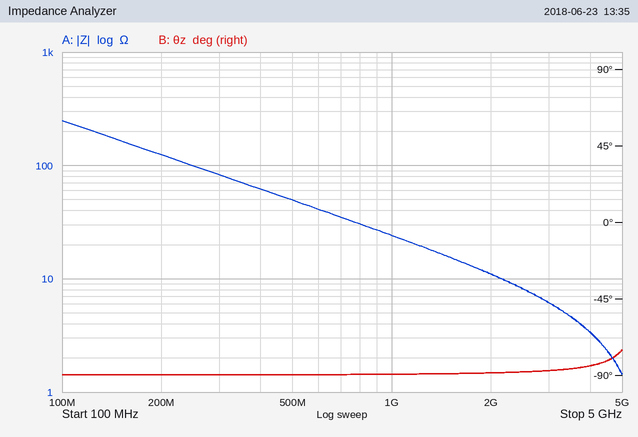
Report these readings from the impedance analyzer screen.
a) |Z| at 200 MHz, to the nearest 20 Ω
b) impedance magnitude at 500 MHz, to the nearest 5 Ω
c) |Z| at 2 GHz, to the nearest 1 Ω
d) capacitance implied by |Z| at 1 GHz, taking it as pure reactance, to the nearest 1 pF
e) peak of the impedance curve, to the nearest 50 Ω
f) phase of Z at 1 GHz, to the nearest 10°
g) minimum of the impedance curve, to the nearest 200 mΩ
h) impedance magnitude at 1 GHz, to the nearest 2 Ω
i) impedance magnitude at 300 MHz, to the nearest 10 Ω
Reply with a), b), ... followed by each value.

a) 120 Ω
b) 50 Ω
c) 11 Ω
d) 7 pF
e) 250 Ω
f) -90°
g) 1.4 Ω
h) 24 Ω
i) 80 Ω
